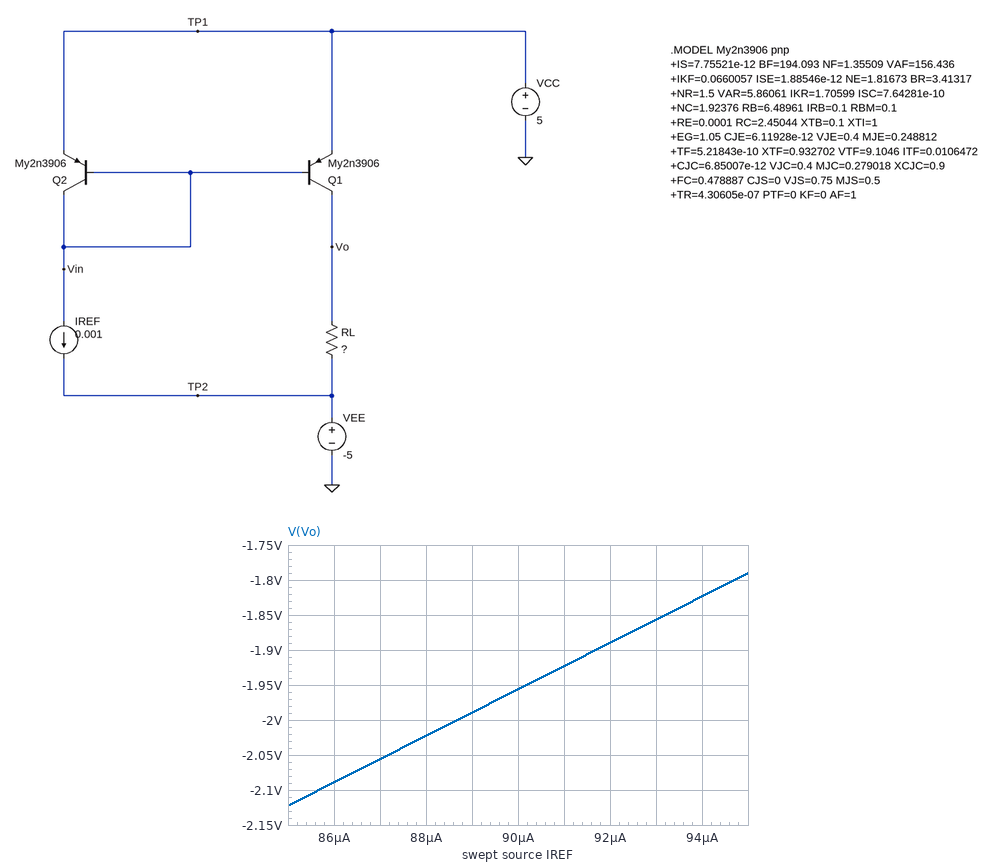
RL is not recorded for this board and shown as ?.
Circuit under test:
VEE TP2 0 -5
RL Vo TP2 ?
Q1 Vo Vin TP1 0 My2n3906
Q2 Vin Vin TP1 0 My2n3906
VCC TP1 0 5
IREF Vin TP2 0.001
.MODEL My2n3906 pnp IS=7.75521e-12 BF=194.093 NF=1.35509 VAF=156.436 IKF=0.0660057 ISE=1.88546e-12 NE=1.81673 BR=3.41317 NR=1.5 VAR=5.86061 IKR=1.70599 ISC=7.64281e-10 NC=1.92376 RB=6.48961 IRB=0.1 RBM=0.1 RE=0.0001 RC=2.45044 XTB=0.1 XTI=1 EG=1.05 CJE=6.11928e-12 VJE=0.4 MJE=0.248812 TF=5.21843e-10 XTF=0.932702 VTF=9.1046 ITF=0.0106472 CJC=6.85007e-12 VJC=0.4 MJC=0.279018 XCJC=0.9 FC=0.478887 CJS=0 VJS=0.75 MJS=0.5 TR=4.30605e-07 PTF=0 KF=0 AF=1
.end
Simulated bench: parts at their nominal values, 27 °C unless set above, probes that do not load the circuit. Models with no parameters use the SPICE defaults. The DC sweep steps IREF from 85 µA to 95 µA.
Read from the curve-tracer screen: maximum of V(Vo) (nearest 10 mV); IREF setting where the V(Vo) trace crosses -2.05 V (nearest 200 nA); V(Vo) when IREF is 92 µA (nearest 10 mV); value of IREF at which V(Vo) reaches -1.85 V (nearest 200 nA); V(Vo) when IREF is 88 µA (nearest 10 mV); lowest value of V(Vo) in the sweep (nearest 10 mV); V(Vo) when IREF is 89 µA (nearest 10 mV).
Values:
-1.79 V
87.2 µA
-1.89 V
93.2 µA
-2.02 V
-2.12 V
-1.99 V
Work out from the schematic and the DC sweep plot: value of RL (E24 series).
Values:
33 kΩ
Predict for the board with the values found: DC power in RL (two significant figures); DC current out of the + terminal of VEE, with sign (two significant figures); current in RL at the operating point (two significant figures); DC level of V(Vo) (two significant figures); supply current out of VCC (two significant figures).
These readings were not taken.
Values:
3.0 mW
-1.3 mA
300 µA
5.0 V
1.3 mA
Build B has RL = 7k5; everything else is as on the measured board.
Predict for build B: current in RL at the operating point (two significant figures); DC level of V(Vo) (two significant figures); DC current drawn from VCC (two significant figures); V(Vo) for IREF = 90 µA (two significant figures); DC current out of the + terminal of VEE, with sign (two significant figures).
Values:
1.0 mA
2.5 V
2.0 mA
-4.3 V
-2.0 mA
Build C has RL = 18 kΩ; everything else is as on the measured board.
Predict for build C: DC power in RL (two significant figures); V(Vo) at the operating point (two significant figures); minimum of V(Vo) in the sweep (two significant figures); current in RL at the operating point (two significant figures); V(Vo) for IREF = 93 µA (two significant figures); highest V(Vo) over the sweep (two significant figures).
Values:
5.5 mW
5.0 V
-3.4 V
550 µA
-3.3 V
-3.2 V
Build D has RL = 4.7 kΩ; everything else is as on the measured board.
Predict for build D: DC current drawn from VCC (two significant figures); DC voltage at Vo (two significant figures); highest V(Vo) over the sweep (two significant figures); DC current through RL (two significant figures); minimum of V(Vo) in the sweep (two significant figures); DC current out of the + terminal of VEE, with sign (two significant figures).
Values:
2.0 mA
-220 mV
-4.5 V
1.0 mA
-4.6 V
-2.0 mA
